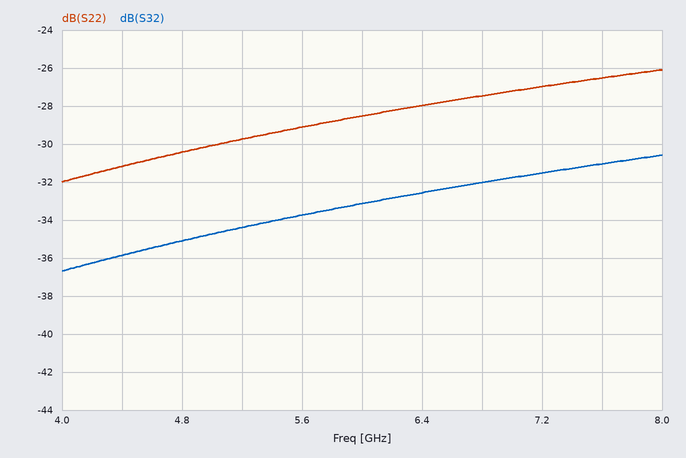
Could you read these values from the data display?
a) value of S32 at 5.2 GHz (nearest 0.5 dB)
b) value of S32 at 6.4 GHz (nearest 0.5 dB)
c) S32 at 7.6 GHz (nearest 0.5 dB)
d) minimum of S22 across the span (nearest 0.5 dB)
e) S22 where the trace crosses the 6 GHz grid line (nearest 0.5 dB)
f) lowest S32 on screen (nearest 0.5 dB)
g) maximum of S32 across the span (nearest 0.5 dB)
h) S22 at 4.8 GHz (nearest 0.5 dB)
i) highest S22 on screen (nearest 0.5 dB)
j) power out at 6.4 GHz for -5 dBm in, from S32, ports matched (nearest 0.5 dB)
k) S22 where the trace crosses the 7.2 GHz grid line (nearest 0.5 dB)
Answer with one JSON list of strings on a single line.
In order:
["-34.5 dB", "-32.5 dB", "-31.0 dB", "-32.0 dB", "-28.5 dB", "-36.5 dB", "-30.5 dB", "-30.5 dB", "-26.0 dB", "-37.5 dBm", "-27.0 dB"]
